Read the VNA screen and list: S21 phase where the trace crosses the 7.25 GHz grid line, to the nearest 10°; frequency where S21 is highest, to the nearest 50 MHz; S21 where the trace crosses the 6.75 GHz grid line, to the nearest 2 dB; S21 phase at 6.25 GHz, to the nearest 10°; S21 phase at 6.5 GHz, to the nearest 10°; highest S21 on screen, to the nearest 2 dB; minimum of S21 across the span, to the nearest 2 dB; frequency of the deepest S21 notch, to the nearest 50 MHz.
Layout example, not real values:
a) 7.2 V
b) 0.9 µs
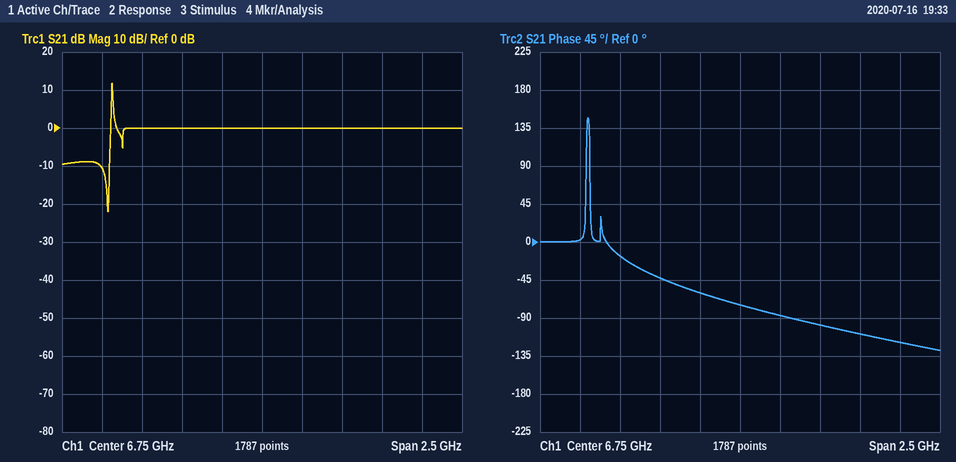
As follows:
a) -100°
b) 5.80 GHz
c) 0 dB
d) -40°
e) -60°
f) 12 dB
g) -22 dB
h) 5.80 GHz
